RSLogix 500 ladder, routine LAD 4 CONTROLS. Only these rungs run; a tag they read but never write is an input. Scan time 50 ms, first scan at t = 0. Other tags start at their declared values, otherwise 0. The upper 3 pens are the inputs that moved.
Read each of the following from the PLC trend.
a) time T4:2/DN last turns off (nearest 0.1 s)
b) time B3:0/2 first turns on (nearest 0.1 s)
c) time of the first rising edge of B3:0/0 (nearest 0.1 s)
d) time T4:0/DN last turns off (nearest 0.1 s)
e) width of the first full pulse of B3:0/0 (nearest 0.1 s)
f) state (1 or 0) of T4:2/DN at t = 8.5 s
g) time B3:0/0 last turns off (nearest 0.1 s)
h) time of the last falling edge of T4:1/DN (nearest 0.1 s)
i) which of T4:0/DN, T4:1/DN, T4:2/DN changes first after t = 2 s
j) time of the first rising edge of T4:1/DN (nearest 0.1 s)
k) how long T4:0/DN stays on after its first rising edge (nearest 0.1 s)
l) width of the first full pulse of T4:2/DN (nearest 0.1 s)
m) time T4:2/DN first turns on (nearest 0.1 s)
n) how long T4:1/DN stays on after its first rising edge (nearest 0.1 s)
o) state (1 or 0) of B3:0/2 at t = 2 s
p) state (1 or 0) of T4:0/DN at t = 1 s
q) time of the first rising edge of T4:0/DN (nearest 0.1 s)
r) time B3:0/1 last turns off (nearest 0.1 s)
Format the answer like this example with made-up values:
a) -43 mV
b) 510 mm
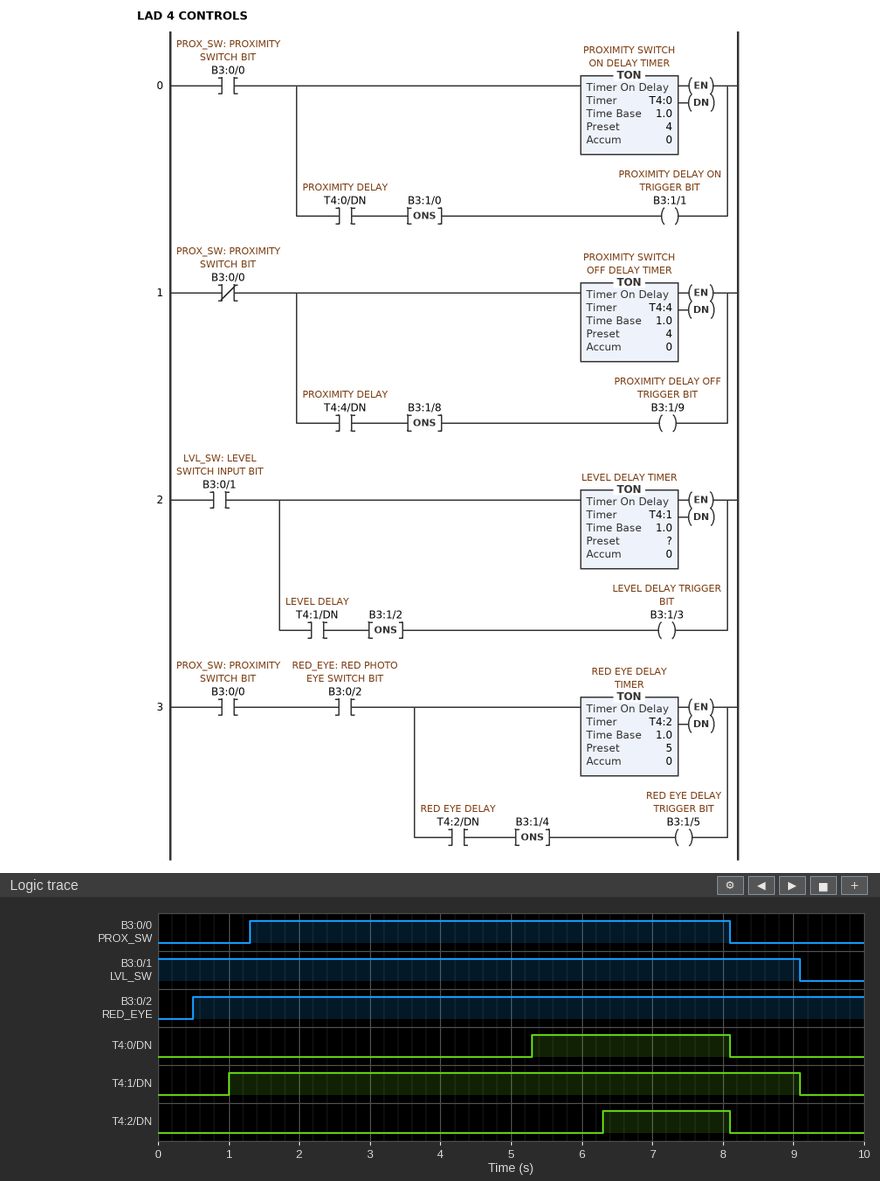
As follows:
a) 8.1 s
b) 0.5 s
c) 1.3 s
d) 8.1 s
e) 6.8 s
f) 0
g) 8.1 s
h) 9.1 s
i) T4:0/DN
j) 1.0 s
k) 2.8 s
l) 1.8 s
m) 6.3 s
n) 8.1 s
o) 1
p) 0
q) 5.3 s
r) 9.1 s
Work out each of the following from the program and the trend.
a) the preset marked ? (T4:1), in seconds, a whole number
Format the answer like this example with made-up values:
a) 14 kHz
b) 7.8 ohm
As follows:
a) 1 s
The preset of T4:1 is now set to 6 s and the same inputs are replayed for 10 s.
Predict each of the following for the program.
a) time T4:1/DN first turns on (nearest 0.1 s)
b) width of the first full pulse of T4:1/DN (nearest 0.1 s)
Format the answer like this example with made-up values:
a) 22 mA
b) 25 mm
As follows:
a) 6.0 s
b) 3.1 s
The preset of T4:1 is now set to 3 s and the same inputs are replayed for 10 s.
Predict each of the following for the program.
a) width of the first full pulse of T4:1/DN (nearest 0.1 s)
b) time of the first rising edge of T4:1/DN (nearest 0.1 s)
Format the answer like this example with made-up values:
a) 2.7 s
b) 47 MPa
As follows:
a) 6.1 s
b) 3.0 s
